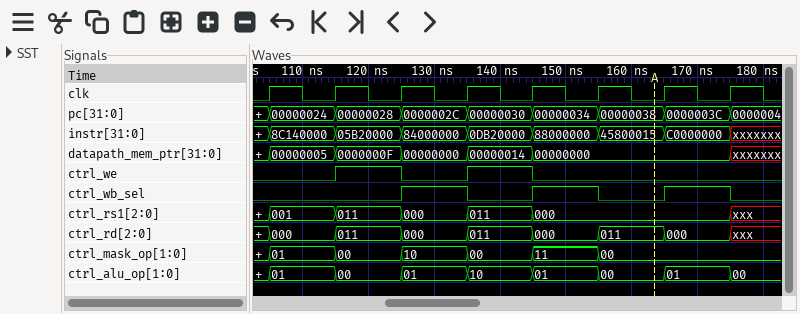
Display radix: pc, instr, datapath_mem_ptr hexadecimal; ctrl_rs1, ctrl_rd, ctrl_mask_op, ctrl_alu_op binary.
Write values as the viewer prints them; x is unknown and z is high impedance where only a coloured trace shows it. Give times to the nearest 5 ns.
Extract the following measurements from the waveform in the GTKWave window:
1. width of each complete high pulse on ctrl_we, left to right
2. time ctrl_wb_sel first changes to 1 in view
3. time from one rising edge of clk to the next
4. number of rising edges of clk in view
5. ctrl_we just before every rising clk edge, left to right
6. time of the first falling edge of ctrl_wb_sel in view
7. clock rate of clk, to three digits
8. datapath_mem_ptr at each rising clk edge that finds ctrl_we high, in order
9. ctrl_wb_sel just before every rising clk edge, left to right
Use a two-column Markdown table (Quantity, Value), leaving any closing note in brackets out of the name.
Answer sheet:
| Quantity | Value |
|---|---|
| width of each complete high pulse on ctrl_we, left to right | 10 ns, 10 ns |
| time ctrl_wb_sel first changes to 1 in view | 125 ns |
| time from one rising edge of clk to the next | 10 ns |
| number of rising edges of clk in view | 8 |
| ctrl_we just before every rising clk edge, left to right | 0 0 1 0 1 0 0 0 |
| time of the first falling edge of ctrl_wb_sel in view | 135 ns |
| clock rate of clk, to three digits | 100 MHz |
| datapath_mem_ptr at each rising clk edge that finds ctrl_we high, in order | 0000000F, 00000014 |
| ctrl_wb_sel just before every rising clk edge, left to right | 0 0 0 1 0 1 0 1 |
